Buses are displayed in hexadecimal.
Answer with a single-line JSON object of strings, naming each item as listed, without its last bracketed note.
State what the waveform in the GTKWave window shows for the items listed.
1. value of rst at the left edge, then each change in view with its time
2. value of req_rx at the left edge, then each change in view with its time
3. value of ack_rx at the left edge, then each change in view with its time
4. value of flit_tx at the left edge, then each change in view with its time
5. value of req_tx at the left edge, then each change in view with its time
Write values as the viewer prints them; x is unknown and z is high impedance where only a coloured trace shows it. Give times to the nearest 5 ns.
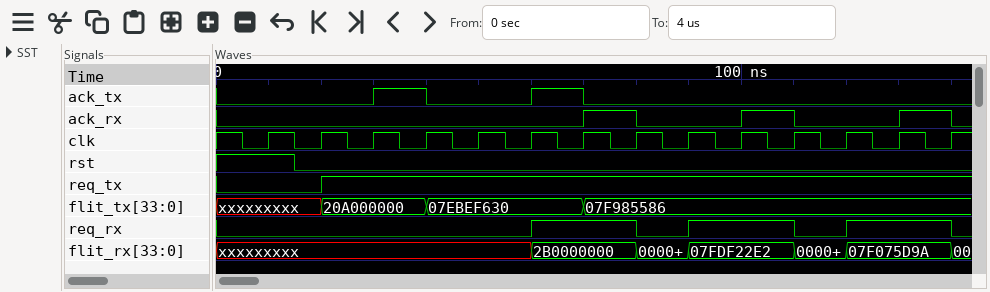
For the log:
{"value of rst at the left edge, then each change in view with its time": "1, 0 at 15 ns", "value of req_rx at the left edge, then each change in view with its time": "0, 1 at 60 ns, 0 at 80 ns, 1 at 90 ns, 0 at 110 ns, 1 at 120 ns, 0 at 140 ns", "value of ack_rx at the left edge, then each change in view with its time": "0, 1 at 70 ns, 0 at 80 ns, 1 at 100 ns, 0 at 110 ns, 1 at 130 ns, 0 at 140 ns", "value of flit_tx at the left edge, then each change in view with its time": "xxxxxxxxx, 20A000000 at 20 ns, 07EBEF630 at 40 ns, 07F985586 at 70 ns", "value of req_tx at the left edge, then each change in view with its time": "0, 1 at 20 ns"}
